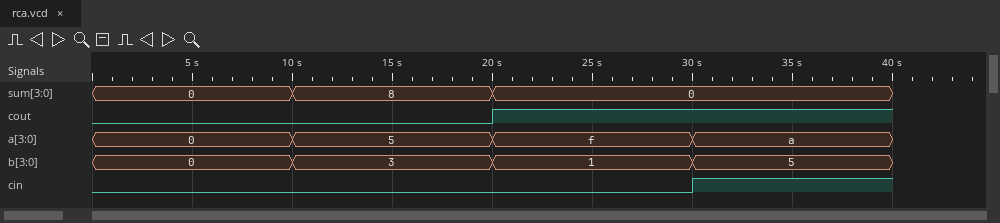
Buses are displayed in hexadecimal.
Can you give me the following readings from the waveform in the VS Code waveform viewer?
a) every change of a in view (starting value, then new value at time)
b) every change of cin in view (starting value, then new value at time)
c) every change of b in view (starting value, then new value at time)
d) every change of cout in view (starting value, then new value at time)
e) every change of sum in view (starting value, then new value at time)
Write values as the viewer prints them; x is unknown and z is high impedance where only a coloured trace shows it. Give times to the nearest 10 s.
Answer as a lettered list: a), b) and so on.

a) 0, 5 at 10 s, f at 20 s, a at 30 s
b) 0, 1 at 30 s
c) 0, 3 at 10 s, 1 at 20 s, 5 at 30 s
d) 0, 1 at 20 s
e) 0, 8 at 10 s, 0 at 20 s
